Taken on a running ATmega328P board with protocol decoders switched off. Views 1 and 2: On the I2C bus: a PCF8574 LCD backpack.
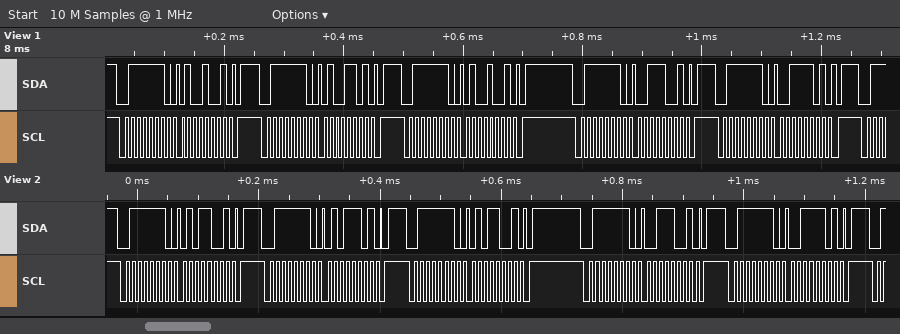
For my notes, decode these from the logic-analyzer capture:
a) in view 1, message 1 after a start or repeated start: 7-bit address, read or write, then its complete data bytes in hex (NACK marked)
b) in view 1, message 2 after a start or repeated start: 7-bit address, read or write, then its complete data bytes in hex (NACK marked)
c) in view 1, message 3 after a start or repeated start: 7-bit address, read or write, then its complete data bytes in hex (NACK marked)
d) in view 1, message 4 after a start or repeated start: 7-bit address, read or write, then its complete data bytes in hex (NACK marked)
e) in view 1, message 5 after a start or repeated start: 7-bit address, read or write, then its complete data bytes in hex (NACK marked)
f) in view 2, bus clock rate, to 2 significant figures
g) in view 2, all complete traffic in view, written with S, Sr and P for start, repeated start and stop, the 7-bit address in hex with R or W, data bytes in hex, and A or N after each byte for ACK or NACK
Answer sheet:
0x3F write: 49
0x3F write: 4D
0x3F write: 49
0x3F write: 39
0x3F write: 3D
100 kHz
S 3FW A 59 A P S 3FW A 5D A P S 3FW A 59 A P S 3FW A 39 A P S 3FW A 3D A P
